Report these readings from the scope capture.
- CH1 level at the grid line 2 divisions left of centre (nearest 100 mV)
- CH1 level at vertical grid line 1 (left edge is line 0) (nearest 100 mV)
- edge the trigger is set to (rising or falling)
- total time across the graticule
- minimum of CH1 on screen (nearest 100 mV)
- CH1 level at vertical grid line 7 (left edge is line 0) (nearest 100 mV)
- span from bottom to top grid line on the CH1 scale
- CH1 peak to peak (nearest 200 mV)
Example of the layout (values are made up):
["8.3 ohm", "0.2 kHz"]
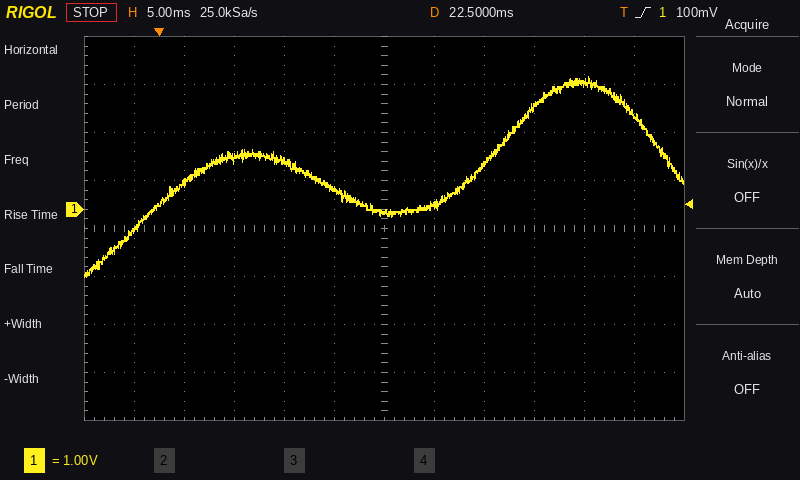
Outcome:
["1.0 V", "-400 mV", "rising", "60 ms", "-1.4 V", "100 mV", "8 V", "4.2 V"]
